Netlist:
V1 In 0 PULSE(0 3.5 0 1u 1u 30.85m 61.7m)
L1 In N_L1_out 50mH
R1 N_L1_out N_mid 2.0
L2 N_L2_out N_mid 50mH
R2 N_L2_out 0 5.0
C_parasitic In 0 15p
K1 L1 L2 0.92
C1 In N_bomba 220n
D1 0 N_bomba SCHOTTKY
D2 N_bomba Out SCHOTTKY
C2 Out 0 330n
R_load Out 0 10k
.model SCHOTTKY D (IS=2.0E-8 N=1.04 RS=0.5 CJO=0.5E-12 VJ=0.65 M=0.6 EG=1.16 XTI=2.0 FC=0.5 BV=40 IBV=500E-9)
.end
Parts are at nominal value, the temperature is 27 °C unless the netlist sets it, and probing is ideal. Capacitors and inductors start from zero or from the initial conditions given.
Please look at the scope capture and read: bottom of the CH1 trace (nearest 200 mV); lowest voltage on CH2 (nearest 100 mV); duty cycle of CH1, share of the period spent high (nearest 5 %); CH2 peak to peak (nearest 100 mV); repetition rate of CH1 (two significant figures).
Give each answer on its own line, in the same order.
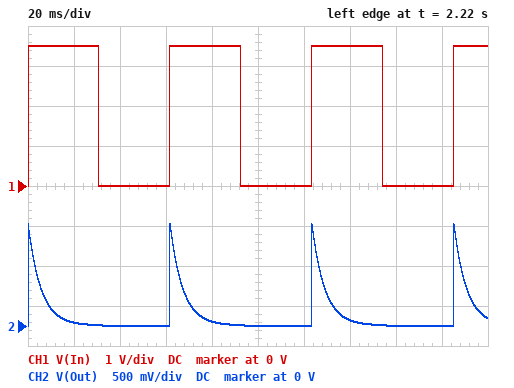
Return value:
0 V
0 V
50 %
1.3 V
16 Hz
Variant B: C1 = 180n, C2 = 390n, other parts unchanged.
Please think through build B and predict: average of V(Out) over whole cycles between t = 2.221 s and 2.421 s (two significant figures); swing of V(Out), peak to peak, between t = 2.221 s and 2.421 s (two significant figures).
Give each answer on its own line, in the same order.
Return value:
97 mV
1.0 V
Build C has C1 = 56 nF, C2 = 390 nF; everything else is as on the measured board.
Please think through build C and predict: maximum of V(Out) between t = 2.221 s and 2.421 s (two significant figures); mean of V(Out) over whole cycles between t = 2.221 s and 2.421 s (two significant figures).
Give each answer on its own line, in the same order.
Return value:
410 mV
31 mV
